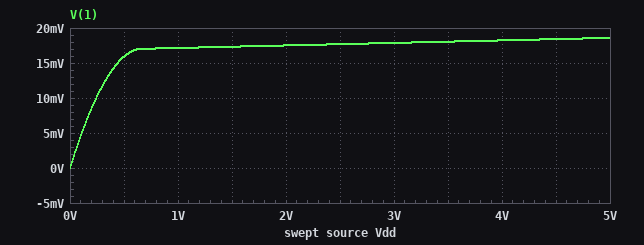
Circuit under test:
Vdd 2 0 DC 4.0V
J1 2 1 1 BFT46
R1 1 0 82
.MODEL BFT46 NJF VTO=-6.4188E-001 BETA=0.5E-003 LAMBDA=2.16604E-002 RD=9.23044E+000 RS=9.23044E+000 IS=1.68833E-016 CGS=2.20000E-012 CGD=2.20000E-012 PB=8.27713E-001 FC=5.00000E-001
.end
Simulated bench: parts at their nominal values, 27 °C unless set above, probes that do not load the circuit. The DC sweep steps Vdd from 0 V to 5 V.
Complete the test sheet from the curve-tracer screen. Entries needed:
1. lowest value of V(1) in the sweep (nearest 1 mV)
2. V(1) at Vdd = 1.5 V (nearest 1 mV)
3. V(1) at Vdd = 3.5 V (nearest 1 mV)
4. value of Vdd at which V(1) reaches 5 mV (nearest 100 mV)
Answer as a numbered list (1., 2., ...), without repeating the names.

1. 0 V
2. 17 mV
3. 18 mV
4. 100 mV
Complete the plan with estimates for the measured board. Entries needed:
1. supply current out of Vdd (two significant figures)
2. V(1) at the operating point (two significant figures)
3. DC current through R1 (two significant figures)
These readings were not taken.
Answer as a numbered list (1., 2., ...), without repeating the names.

1. 220 µA
2. 18 mV
3. 220 µA
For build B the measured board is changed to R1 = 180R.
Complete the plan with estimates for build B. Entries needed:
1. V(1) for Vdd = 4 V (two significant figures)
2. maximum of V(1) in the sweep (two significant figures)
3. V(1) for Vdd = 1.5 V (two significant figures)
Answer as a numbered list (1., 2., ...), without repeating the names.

1. 40 mV
2. 41 mV
3. 38 mV
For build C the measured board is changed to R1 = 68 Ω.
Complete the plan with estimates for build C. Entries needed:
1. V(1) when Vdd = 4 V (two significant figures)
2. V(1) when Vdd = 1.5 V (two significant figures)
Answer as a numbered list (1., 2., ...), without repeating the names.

1. 15 mV
2. 14 mV
